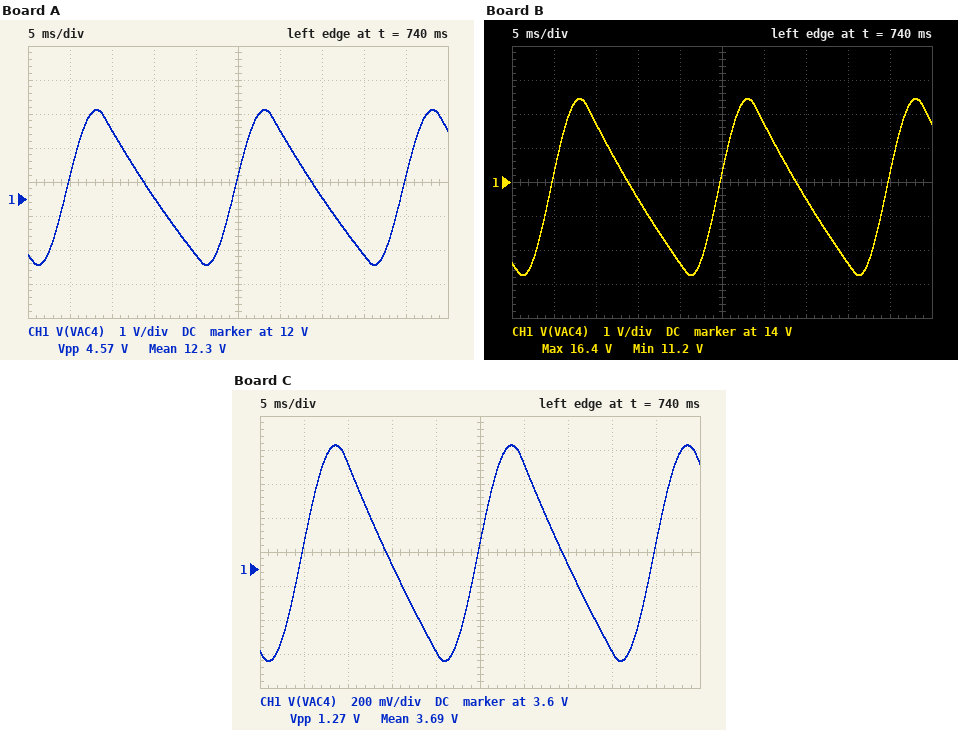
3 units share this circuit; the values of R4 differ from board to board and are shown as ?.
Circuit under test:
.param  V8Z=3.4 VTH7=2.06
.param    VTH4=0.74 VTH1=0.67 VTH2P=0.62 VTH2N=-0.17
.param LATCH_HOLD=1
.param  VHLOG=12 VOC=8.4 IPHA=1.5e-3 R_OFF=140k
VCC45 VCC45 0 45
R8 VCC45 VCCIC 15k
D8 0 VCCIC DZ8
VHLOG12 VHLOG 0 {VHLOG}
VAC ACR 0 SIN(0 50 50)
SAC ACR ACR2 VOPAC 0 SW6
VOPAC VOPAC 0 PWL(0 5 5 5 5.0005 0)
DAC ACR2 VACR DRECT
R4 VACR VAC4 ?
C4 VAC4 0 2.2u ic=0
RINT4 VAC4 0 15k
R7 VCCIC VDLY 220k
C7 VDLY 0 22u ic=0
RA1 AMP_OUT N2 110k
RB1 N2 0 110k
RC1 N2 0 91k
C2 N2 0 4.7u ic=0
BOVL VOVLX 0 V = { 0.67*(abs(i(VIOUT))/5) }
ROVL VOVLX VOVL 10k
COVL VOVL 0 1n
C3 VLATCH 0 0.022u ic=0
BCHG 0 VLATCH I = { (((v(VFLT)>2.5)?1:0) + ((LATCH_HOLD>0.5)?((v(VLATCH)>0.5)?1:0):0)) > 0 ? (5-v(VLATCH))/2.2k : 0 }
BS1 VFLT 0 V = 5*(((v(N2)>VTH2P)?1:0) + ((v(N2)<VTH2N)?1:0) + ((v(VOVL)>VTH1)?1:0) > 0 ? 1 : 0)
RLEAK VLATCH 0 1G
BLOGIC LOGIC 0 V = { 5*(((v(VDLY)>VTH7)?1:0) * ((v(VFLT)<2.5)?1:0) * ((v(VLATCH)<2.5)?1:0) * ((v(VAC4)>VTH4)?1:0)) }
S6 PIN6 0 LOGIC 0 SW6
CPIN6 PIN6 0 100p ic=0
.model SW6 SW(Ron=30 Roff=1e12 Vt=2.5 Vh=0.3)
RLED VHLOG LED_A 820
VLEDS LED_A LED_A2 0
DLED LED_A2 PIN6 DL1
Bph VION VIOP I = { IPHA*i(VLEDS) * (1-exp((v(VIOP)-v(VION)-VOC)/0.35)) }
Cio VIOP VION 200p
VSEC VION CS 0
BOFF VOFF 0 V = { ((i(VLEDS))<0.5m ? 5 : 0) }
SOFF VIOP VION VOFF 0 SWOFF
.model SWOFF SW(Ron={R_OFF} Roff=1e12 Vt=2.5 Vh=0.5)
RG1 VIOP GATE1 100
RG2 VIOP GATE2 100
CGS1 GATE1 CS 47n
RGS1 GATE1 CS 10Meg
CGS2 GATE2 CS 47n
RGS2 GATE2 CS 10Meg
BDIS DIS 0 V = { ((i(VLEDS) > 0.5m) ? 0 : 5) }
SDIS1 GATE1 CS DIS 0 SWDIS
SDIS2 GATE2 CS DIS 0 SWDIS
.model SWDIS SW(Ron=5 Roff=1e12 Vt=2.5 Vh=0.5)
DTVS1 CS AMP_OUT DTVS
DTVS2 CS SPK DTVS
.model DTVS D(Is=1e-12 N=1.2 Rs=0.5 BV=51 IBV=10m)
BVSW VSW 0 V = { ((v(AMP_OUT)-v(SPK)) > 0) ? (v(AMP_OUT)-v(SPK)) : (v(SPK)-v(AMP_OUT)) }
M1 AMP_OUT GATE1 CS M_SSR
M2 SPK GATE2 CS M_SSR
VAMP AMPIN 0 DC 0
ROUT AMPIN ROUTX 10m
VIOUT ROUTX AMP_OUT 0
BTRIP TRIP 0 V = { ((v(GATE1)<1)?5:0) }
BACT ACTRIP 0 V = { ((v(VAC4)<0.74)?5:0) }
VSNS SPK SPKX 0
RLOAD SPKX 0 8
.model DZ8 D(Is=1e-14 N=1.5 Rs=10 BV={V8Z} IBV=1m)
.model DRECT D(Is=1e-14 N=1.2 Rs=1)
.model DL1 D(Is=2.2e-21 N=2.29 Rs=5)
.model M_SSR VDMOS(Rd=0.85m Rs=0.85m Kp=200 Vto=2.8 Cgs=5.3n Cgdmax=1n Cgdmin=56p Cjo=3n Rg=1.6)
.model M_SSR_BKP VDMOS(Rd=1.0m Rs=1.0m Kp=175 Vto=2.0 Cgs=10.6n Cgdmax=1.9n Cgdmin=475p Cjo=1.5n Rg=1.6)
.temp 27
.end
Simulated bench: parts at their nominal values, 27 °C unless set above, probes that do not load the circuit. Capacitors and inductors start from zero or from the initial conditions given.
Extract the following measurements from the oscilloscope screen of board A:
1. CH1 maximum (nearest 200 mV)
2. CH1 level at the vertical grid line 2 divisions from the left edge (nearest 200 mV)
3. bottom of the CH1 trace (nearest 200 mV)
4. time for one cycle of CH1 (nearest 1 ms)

14.6 V
14.0 V
10.0 V
20 ms
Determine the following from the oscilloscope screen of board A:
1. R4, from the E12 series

12 kΩ
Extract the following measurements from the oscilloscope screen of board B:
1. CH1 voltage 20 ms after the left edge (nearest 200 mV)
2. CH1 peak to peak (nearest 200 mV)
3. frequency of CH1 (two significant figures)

11.6 V
5.2 V
50 Hz
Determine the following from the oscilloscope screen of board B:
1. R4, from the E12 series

10 kΩ
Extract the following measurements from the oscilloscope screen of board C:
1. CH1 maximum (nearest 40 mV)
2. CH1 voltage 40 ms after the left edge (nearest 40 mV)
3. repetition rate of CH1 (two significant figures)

4.32 V
3.12 V
50 Hz
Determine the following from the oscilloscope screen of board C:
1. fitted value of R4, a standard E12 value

56 kΩ
